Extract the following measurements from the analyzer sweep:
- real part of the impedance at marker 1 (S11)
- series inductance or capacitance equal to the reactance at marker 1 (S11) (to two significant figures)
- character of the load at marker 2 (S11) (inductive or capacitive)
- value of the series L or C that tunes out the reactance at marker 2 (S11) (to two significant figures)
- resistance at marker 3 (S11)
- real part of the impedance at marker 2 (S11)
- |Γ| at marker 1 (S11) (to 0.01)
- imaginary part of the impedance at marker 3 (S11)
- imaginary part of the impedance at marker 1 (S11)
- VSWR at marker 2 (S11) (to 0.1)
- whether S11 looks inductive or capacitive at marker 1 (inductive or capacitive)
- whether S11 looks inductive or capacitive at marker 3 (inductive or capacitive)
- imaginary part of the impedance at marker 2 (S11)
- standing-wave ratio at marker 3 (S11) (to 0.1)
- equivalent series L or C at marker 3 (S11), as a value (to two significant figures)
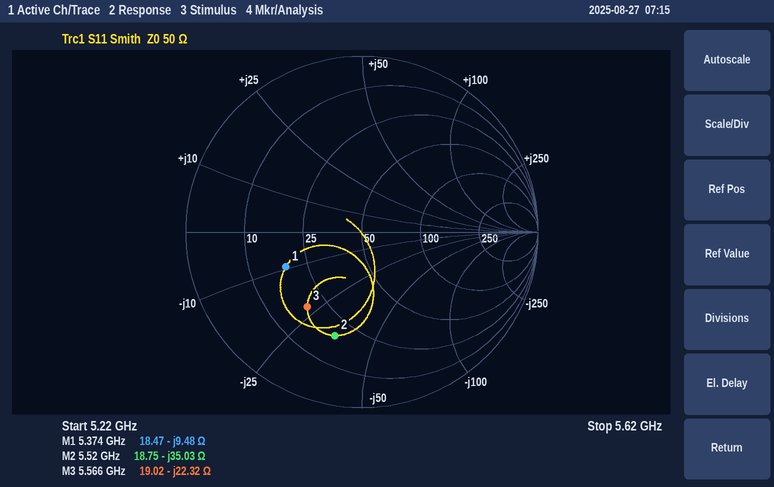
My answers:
18.47 Ω
3.1 pF
capacitive
1.0 nH
19.02 Ω
18.75 Ω
0.48
-22.32 Ω
-9.48 Ω
4.1
capacitive
capacitive
-35.03 Ω
3.2
1.3 pF
